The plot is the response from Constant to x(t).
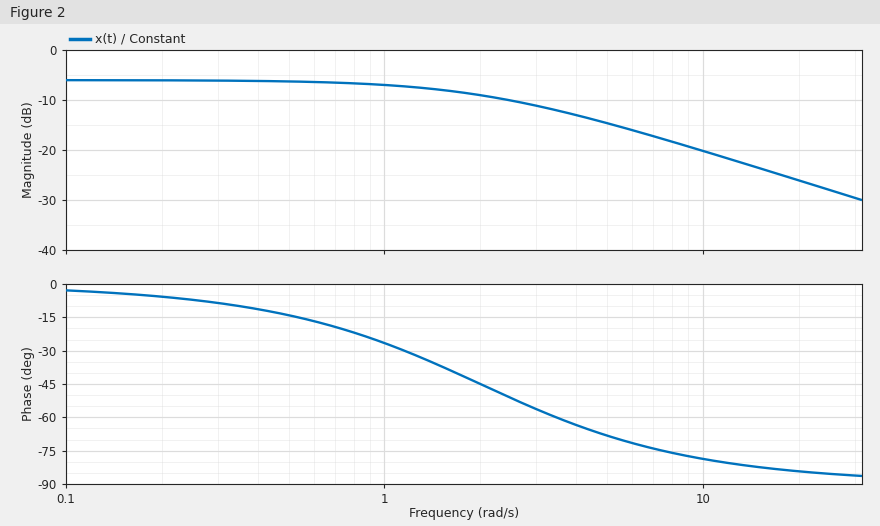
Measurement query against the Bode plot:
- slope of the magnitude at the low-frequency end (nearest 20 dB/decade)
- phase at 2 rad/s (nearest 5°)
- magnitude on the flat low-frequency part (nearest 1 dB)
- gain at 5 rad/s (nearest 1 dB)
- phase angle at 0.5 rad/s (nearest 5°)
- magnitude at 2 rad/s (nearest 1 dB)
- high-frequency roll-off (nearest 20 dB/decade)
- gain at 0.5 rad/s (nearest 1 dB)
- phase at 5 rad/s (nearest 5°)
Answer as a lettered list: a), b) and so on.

a) 0 dB/decade
b) -45°
c) -6 dB
d) -15 dB
e) -15°
f) -9 dB
g) -20 dB/decade
h) -6 dB
i) -70°
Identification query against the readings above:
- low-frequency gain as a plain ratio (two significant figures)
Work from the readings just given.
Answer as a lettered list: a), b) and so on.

a) 0.50
